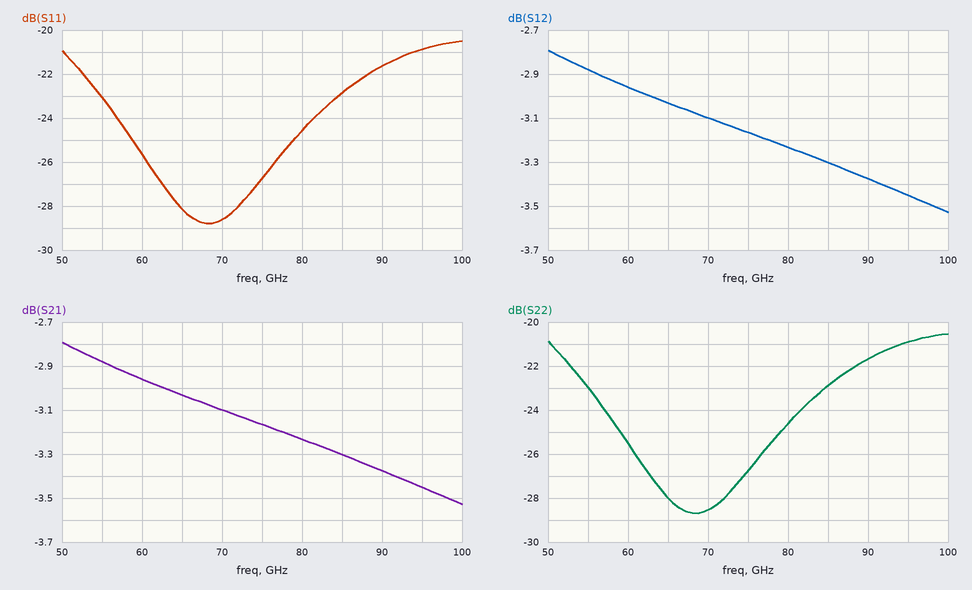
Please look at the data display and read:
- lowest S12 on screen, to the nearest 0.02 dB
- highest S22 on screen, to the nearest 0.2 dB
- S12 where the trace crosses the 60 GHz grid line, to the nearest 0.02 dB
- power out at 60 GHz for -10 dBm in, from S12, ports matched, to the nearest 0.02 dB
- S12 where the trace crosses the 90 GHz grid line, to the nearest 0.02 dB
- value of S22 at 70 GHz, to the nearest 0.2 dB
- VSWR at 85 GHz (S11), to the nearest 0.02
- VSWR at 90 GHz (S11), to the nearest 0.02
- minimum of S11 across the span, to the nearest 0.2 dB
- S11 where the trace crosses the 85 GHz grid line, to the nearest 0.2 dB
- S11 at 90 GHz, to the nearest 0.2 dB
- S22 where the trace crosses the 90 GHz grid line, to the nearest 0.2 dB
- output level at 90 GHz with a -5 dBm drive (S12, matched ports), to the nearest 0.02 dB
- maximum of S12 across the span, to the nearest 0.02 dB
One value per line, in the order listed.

-3.52 dB
-20.6 dB
-2.96 dB
-12.96 dBm
-3.38 dB
-28.6 dB
1.16
1.18
-28.8 dB
-22.8 dB
-21.6 dB
-21.6 dB
-8.38 dBm
-2.80 dB
